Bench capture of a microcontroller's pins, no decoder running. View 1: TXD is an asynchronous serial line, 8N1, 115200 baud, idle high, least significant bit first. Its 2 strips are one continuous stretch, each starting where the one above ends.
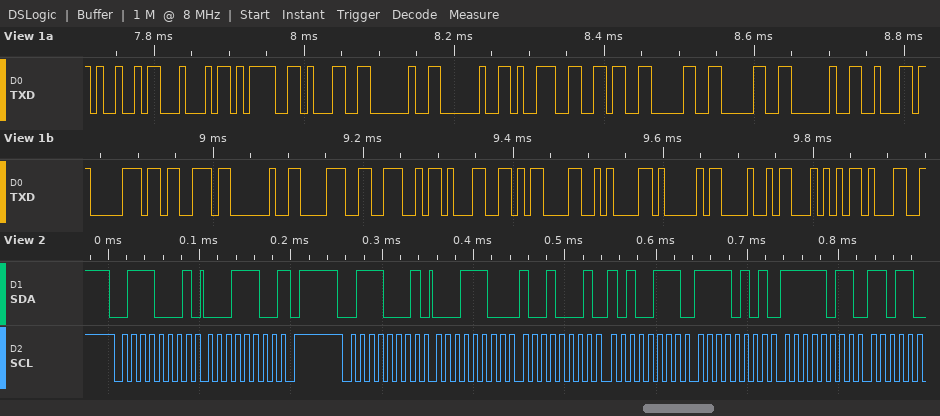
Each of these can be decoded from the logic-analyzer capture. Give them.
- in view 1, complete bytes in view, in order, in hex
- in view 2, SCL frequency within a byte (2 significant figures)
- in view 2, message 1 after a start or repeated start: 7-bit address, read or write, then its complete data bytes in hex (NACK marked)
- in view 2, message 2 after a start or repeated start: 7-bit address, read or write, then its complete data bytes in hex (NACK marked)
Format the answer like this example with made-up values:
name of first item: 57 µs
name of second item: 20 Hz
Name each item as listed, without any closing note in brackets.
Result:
in view 1, complete bytes in view, in order, in hex: 49 44 3D 31 20 20 39 36 30 30 20 62 70 73 20 38 4E 31 0D 0A 41 48 54 31
in view 2, SCL frequency within a byte: 100 kHz
in view 2, message 1 after a start or repeated start: 7-bit address, read or write, then its complete data bytes in hex: 0x38 read: 1C NACK
in view 2, message 2 after a start or repeated start: 7-bit address, read or write, then its complete data bytes in hex: 0x38 read: 1C 91 A7 F5 FB
